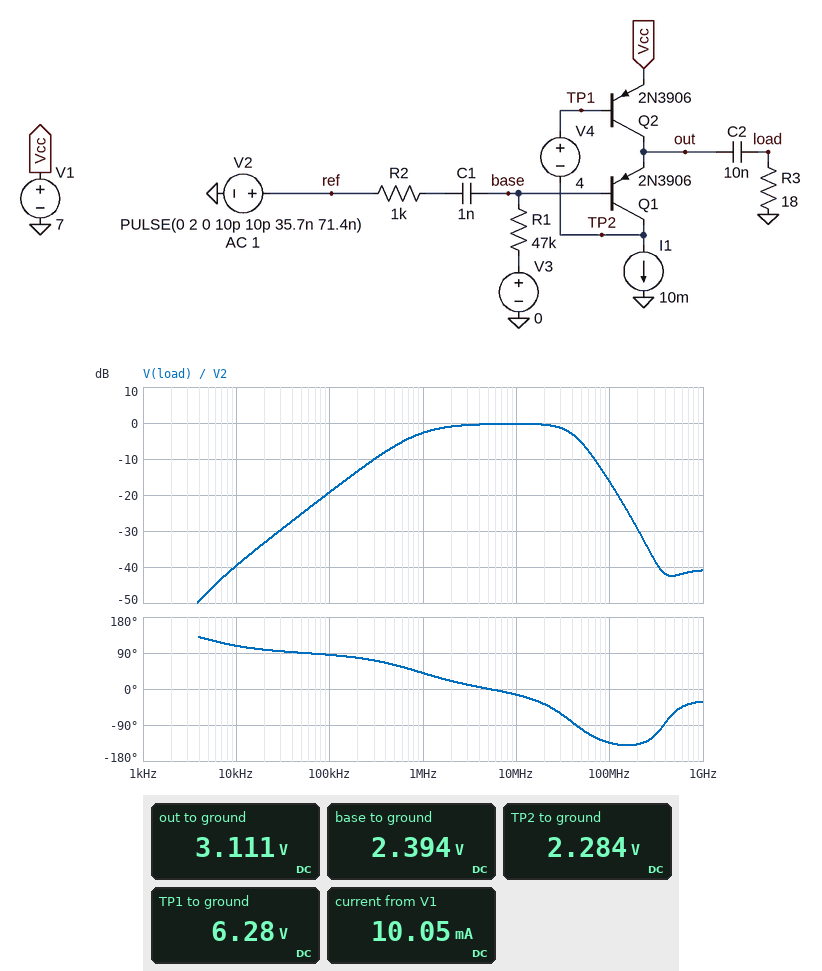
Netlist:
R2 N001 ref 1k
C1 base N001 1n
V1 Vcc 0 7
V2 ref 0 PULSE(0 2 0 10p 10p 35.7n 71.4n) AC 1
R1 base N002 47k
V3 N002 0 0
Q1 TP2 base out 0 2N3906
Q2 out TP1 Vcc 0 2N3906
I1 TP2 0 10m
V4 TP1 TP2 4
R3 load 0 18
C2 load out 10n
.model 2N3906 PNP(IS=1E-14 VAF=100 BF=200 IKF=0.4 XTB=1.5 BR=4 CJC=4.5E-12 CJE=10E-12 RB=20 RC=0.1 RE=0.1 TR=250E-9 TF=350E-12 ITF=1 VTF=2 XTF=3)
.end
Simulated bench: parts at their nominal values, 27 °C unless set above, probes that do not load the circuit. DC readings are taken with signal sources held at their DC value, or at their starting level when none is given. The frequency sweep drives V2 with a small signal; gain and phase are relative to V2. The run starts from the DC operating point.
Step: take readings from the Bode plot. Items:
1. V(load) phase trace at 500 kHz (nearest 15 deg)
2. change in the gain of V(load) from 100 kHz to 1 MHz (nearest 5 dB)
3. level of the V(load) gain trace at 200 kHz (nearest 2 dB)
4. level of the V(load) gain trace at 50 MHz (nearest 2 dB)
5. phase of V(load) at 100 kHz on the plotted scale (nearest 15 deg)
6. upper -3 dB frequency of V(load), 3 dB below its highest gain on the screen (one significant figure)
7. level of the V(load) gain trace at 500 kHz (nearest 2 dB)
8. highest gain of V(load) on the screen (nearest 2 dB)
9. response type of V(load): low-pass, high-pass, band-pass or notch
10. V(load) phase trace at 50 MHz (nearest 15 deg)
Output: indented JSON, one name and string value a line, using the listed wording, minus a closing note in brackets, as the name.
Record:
{
  "V(load) phase trace at 500 kHz": "60 deg",
  "change in the gain of V(load) from 100 kHz to 1 MHz": "15 dB",
  "level of the V(load) gain trace at 200 kHz": "-14 dB",
  "level of the V(load) gain trace at 50 MHz": "-6 dB",
  "phase of V(load) at 100 kHz on the plotted scale": "90 deg",
  "upper -3 dB frequency of V(load), 3 dB below its highest gain on the screen": "40 MHz",
  "level of the V(load) gain trace at 500 kHz": "-6 dB",
  "highest gain of V(load) on the screen": "0 dB",
  "response type of V(load): low-pass, high-pass, band-pass or notch": "band-pass",
  "V(load) phase trace at 50 MHz": "-105 deg"
}
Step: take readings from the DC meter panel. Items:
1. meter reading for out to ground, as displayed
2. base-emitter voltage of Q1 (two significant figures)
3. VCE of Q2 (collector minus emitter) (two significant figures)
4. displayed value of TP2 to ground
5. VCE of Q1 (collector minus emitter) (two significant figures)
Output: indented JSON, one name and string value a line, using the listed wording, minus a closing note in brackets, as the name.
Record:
{
  "meter reading for out to ground, as displayed": "3.111 V",
  "base-emitter voltage of Q1": "-720 mV",
  "VCE of Q2 (collector minus emitter)": "-3.9 V",
  "displayed value of TP2 to ground": "2.284 V",
  "VCE of Q1 (collector minus emitter)": "-830 mV"
}
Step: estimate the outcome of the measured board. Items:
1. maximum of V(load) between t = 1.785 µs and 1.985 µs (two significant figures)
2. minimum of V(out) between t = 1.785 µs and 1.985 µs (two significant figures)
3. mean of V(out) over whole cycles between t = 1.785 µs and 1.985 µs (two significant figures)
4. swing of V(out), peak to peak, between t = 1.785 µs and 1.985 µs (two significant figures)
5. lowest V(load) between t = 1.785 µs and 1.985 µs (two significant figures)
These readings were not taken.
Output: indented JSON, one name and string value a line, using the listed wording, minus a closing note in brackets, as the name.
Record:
{
  "maximum of V(load) between t = 1.785 µs and 1.985 µs": "1.2 V",
  "minimum of V(out) between t = 1.785 µs and 1.985 µs": "3.8 V",
  "mean of V(out) over whole cycles between t = 1.785 µs and 1.985 µs": "4.1 V",
  "swing of V(out), peak to peak, between t = 1.785 µs and 1.985 µs": "1.4 V",
  "lowest V(load) between t = 1.785 µs and 1.985 µs": "-290 mV"
}
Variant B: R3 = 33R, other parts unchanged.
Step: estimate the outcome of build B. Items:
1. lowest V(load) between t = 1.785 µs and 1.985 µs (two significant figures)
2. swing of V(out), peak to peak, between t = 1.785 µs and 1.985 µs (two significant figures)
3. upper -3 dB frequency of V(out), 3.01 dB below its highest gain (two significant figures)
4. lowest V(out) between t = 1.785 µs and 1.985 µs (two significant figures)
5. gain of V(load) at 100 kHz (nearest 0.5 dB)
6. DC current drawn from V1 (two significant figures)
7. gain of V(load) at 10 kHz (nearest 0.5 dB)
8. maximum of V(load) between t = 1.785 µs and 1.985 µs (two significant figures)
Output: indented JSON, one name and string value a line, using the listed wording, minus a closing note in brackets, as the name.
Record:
{
  "lowest V(load) between t = 1.785 µs and 1.985 µs": "-450 mV",
  "swing of V(out), peak to peak, between t = 1.785 µs and 1.985 µs": "1.6 V",
  "upper -3 dB frequency of V(out), 3.01 dB below its highest gain": "43 MHz",
  "lowest V(out) between t = 1.785 µs and 1.985 µs": "3.6 V",
  "gain of V(load) at 100 kHz": "-14.0 dB",
  "DC current drawn from V1": "10 mA",
  "gain of V(load) at 10 kHz": "-34.5 dB",
  "maximum of V(load) between t = 1.785 µs and 1.985 µs": "1.1 V"
}
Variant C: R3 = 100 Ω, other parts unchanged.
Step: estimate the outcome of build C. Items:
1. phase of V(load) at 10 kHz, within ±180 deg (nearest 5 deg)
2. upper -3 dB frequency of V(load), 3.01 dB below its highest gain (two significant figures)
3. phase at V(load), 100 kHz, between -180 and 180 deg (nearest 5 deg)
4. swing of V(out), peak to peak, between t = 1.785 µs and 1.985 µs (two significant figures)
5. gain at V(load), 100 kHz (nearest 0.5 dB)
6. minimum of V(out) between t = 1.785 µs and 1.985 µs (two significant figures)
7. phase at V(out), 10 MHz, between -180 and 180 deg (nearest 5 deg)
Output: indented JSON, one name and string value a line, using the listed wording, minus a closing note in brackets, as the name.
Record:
{
  "phase of V(load) at 10 kHz, within ±180 deg": "105 deg",
  "upper -3 dB frequency of V(load), 3.01 dB below its highest gain": "44 MHz",
  "phase at V(load), 100 kHz, between -180 and 180 deg": "60 deg",
  "swing of V(out), peak to peak, between t = 1.785 µs and 1.985 µs": "2.0 V",
  "gain at V(load), 100 kHz": "-5.5 dB",
  "minimum of V(out) between t = 1.785 µs and 1.985 µs": "3.1 V",
  "phase at V(out), 10 MHz, between -180 and 180 deg": "-15 deg"
}
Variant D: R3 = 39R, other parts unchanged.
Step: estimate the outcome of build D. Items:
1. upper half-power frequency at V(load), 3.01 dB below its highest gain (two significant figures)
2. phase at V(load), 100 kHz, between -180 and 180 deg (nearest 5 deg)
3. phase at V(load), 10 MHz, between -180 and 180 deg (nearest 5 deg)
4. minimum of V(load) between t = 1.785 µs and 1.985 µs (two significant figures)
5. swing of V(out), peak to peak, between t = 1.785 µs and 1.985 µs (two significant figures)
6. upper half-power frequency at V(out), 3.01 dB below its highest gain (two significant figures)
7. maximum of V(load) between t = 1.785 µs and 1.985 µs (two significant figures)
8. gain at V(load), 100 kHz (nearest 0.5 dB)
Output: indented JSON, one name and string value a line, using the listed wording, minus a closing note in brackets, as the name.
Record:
{
  "upper half-power frequency at V(load), 3.01 dB below its highest gain": "44 MHz",
  "phase at V(load), 100 kHz, between -180 and 180 deg": "80 deg",
  "phase at V(load), 10 MHz, between -180 and 180 deg": "-15 deg",
  "minimum of V(load) between t = 1.785 µs and 1.985 µs": "-510 mV",
  "swing of V(out), peak to peak, between t = 1.785 µs and 1.985 µs": "1.6 V",
  "upper half-power frequency at V(out), 3.01 dB below its highest gain": "43 MHz",
  "maximum of V(load) between t = 1.785 µs and 1.985 µs": "1.1 V",
  "gain at V(load), 100 kHz": "-12.5 dB"
}
